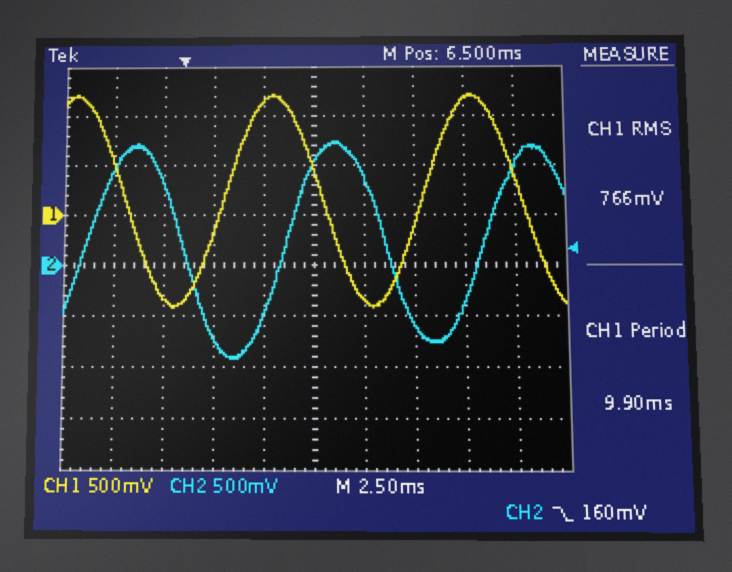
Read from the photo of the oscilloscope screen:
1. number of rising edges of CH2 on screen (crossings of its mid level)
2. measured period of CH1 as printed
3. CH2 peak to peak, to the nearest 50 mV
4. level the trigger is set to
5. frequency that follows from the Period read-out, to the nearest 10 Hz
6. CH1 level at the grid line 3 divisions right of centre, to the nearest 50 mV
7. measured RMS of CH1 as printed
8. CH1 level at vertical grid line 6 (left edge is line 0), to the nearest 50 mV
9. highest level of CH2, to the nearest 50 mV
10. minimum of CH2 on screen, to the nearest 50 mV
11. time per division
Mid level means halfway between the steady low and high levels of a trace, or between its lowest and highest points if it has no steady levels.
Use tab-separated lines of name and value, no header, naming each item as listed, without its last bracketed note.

number of rising edges of CH2 on screen	3
measured period of CH1 as printed	9.90 ms
CH2 peak to peak, to the nearest 50 mV	2.15 V
level the trigger is set to	160 mV
frequency that follows from the Period read-out, to the nearest 10 Hz	100 Hz
CH1 level at the grid line 3 divisions right of centre, to the nearest 50 mV	1.15 V
measured RMS of CH1 as printed	766 mV
CH1 level at vertical grid line 6 (left edge is line 0), to the nearest 50 mV	-850 mV
highest level of CH2, to the nearest 50 mV	1.25 V
minimum of CH2 on screen, to the nearest 50 mV	-900 mV
time per division	2.5 ms
